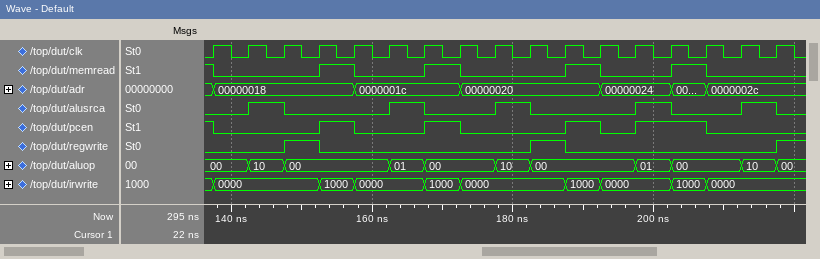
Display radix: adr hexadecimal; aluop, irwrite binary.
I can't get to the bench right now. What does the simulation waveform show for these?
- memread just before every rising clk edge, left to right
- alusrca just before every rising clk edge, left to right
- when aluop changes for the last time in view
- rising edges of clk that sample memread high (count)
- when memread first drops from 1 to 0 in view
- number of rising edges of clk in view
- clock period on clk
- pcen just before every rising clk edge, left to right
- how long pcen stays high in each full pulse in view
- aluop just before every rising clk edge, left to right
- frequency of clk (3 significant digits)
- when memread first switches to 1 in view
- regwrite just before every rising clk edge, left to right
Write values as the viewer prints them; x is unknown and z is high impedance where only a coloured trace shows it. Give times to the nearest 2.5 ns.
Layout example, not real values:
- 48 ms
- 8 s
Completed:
- 1 0 0 0 1 0 0 1 0 0 0 1 0 0 1 0 0
- 0 0 1 0 0 0 1 0 0 1 0 0 0 1 0 0 1
- 217.5 ns
- 5
- 137.5 ns
- 17
- 5 ns
- 1 0 0 0 1 0 0 1 0 0 0 1 0 1 1 0 0
- 5 ns, 5 ns, 5 ns, 10 ns
- 00, 00, 10, 00, 00, 00, 01, 00, 00, 10, 00, 00, 00, 01, 00, 00, 10
- 200 MHz
- 152.5 ns
- 0 0 0 1 0 0 0 0 0 0 1 0 0 0 0 0 0
